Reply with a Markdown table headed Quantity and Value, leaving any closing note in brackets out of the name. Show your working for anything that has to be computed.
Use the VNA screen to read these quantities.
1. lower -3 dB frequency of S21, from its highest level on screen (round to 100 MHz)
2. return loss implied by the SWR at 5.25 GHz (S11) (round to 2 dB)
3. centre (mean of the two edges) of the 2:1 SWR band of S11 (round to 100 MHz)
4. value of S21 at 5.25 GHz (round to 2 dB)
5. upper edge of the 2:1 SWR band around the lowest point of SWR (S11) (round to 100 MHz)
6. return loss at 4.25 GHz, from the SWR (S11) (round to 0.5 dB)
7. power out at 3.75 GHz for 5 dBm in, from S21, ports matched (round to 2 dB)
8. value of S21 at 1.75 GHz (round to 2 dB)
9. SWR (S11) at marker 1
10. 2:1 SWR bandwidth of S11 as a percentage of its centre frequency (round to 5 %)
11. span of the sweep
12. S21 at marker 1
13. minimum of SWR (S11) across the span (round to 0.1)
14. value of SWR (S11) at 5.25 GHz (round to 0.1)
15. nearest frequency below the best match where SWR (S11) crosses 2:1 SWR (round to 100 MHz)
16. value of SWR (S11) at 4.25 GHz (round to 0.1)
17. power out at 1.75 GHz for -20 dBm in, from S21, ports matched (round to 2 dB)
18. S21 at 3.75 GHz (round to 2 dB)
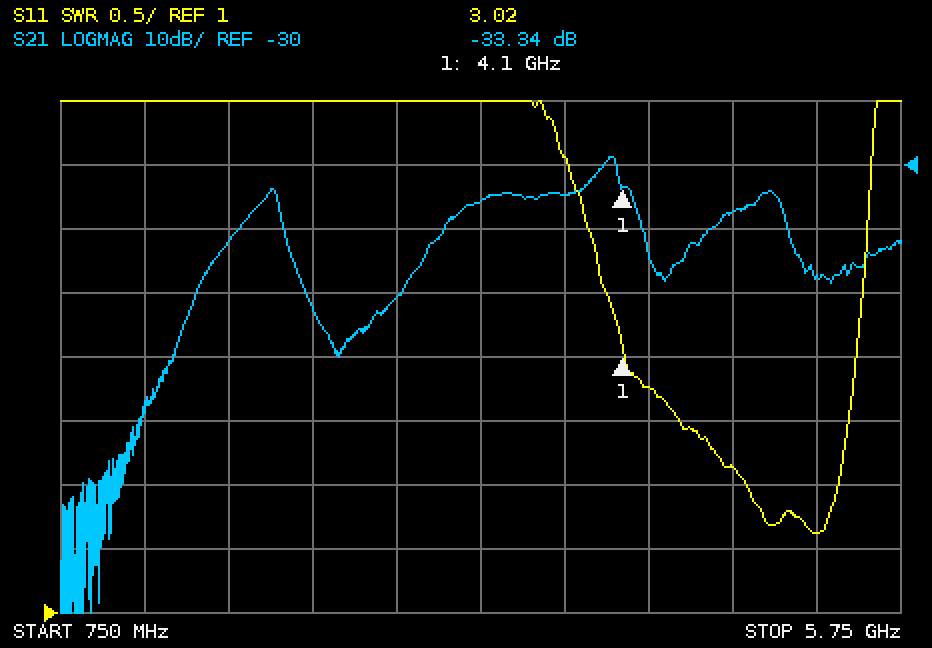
| Quantity | Value |
|---|---|
| lower -3 dB frequency of S21, from its highest level on screen | 3.9 GHz |
| return loss implied by the SWR at 5.25 GHz (S11) | −20 log10((1.6 − 1)/(1.6 + 1)) ≈ 12.7 dB, so 12 dB to the nearest 2 dB |
| centre (mean of the two edges) of the 2:1 SWR band of S11 | 5.1 GHz |
| value of S21 at 5.25 GHz | -48 dB |
| upper edge of the 2:1 SWR band around the lowest point of SWR (S11) | 5.4 GHz |
| return loss at 4.25 GHz, from the SWR (S11) | −20 log10((2.8 − 1)/(2.8 + 1)) ≈ 6.5 dB |
| power out at 3.75 GHz for 5 dBm in, from S21, ports matched | 5 dBm + (-34 dB) = -30 dBm |
| value of S21 at 1.75 GHz | -42 dB |
| SWR (S11) at marker 1 | 3.02 |
| 2:1 SWR bandwidth of S11 as a percentage of its centre frequency | 600 MHz / 5.1 GHz ≈ 11.8 %, so 10 % to the nearest 5 % |
| span of the sweep | 5 GHz |
| S21 at marker 1 | -33.34 dB |
| minimum of SWR (S11) across the span | 1.6 |
| value of SWR (S11) at 5.25 GHz | 1.6 |
| nearest frequency below the best match where SWR (S11) crosses 2:1 SWR | 4.8 GHz |
| value of SWR (S11) at 4.25 GHz | 2.8 |
| power out at 1.75 GHz for -20 dBm in, from S21, ports matched | -20 dBm + (-42 dB) = -62 dBm |
| S21 at 3.75 GHz | -34 dB |
